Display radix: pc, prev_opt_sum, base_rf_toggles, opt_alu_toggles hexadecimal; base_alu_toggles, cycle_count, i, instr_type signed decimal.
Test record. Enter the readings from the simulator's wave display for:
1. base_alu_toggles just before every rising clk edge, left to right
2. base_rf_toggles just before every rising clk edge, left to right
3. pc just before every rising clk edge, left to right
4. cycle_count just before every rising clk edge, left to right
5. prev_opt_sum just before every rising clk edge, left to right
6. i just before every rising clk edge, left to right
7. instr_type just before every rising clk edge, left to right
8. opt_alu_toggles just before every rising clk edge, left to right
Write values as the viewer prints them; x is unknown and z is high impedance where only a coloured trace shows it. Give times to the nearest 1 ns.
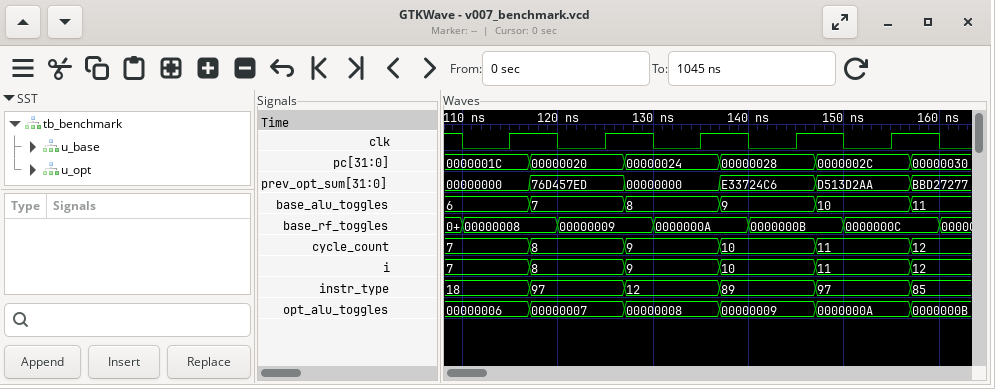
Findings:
6, 7, 8, 9, 10
00000008, 00000009, 0000000A, 0000000B, 0000000C
0000001C, 00000020, 00000024, 00000028, 0000002C
7, 8, 9, 10, 11
00000000, 76D457ED, 00000000, E33724C6, D513D2AA
7, 8, 9, 10, 11
18, 97, 12, 89, 97
00000006, 00000007, 00000008, 00000009, 0000000A
